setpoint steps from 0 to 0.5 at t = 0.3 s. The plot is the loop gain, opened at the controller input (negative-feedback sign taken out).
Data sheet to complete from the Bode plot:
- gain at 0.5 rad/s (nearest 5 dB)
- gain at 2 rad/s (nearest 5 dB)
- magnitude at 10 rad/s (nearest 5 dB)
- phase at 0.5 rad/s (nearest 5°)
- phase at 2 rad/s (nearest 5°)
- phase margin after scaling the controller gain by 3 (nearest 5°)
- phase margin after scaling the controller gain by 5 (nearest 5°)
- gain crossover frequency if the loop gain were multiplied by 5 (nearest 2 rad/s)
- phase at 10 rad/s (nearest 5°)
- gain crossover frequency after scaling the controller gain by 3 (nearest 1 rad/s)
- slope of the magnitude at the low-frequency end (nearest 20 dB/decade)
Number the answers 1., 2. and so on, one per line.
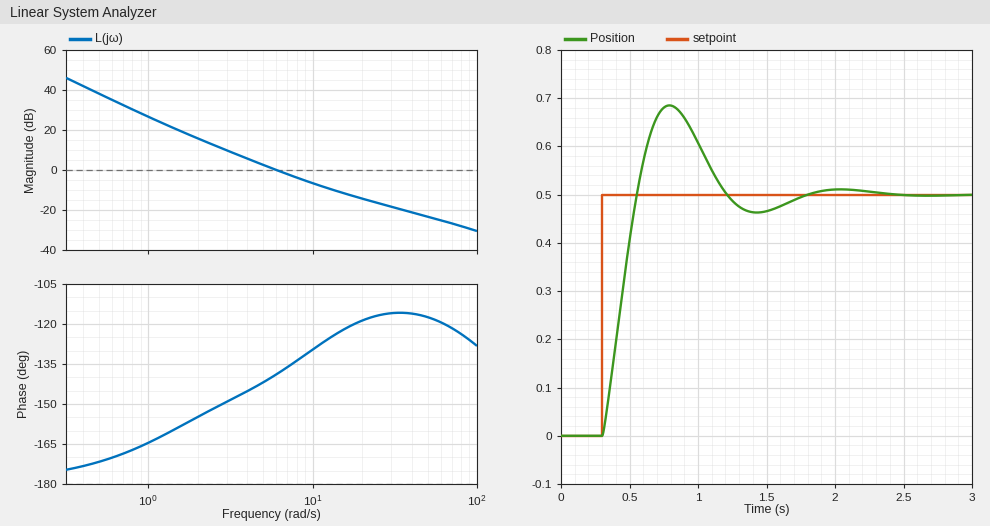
1. 40 dB
2. 15 dB
3. -5 dB
4. -170°
5. -155°
6. 55°
7. 60°
8. 20 rad/s
9. -130°
10. 13 rad/s
11. -40 dB/decade
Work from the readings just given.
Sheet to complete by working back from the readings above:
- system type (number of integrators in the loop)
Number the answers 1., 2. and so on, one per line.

1. 2
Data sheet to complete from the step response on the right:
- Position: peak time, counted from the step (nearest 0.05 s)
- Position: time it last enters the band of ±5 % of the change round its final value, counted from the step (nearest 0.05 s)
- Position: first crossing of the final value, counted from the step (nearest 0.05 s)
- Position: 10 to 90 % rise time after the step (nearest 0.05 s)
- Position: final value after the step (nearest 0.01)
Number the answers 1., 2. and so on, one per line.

1. 0.50 s
2. 1.30 s
3. 0.25 s
4. 0.20 s
5. 0.50
